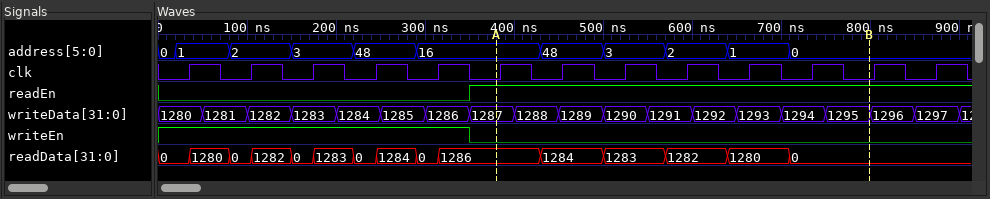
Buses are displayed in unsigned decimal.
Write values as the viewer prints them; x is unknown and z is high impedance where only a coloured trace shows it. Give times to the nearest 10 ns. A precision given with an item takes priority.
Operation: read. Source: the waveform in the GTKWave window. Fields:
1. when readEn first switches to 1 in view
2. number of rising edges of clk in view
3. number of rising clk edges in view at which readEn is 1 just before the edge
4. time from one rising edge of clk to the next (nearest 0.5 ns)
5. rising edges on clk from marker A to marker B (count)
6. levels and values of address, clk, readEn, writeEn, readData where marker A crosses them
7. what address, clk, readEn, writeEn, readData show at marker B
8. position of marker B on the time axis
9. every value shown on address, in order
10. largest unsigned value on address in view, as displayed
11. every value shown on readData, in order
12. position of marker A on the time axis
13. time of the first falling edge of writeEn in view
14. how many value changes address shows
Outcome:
350 ns
13
8
70 ns
6
address=16, clk=0, readEn=1, writeEn=0, readData=1286
address=0, clk=0, readEn=1, writeEn=0, readData=0
800 ns
0, 1, 2, 3, 48, 16, 48, 3, 2, 1, 0
48
0, 1280, 0, 1282, 0, 1283, 0, 1284, 0, 1286, 1284, 1283, 1282, 1280, 0
380 ns
350 ns
10
